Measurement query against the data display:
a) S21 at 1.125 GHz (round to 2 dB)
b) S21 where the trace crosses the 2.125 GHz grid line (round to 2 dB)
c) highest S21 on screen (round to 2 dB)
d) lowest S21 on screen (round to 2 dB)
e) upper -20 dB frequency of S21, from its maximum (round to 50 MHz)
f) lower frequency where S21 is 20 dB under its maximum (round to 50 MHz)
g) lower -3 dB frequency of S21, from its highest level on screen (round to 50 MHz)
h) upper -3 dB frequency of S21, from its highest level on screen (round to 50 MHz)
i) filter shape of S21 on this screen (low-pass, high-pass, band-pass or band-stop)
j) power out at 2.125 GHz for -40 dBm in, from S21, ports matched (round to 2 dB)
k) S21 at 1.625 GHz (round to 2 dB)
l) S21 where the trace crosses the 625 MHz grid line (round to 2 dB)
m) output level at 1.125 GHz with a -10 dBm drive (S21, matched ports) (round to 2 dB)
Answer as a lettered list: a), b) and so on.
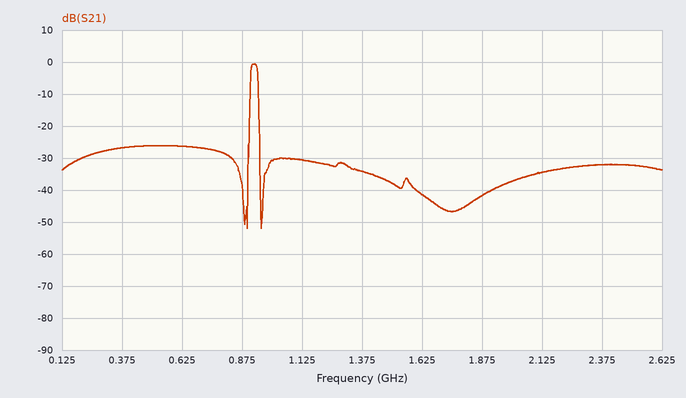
a) -30 dB
b) -34 dB
c) 0 dB
d) -52 dB
e) 950 MHz
f) 900 MHz
g) 900 MHz
h) 950 MHz
i) band-pass
j) -74 dBm
k) -42 dB
l) -26 dB
m) -40 dBm
